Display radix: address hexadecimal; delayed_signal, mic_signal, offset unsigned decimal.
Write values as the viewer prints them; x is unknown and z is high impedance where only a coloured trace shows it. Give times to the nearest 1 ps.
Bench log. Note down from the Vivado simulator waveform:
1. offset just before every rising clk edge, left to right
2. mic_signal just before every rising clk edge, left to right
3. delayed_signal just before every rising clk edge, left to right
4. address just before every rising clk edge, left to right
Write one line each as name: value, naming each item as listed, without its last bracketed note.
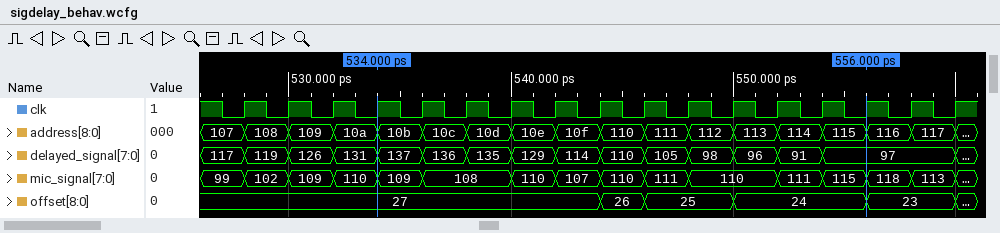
offset just before every rising clk edge, left to right: 27, 27, 27, 27, 27, 27, 27, 27, 27, 26, 25, 25, 24, 24, 24, 23, 23
mic_signal just before every rising clk edge, left to right: 99, 102, 109, 110, 109, 108, 108, 110, 107, 110, 111, 110, 110, 111, 115, 118, 113
delayed_signal just before every rising clk edge, left to right: 117, 119, 126, 131, 137, 136, 135, 129, 114, 110, 105, 98, 96, 91, 97, 97, 97
address just before every rising clk edge, left to right: 107, 108, 109, 10a, 10b, 10c, 10d, 10e, 10f, 110, 111, 112, 113, 114, 115, 116, 117
